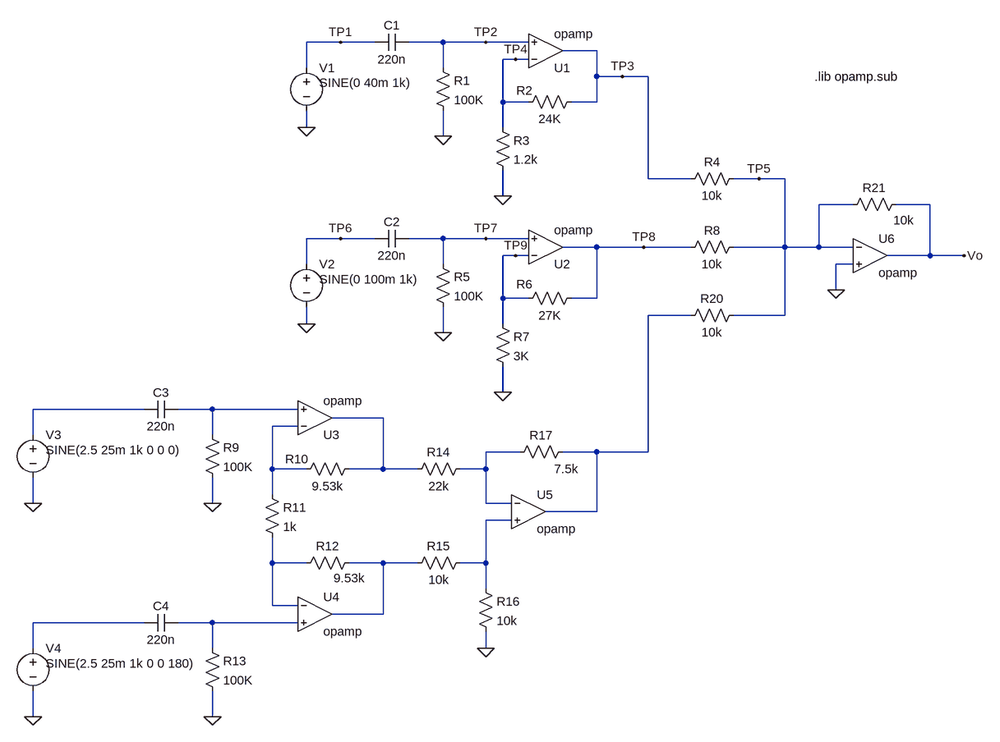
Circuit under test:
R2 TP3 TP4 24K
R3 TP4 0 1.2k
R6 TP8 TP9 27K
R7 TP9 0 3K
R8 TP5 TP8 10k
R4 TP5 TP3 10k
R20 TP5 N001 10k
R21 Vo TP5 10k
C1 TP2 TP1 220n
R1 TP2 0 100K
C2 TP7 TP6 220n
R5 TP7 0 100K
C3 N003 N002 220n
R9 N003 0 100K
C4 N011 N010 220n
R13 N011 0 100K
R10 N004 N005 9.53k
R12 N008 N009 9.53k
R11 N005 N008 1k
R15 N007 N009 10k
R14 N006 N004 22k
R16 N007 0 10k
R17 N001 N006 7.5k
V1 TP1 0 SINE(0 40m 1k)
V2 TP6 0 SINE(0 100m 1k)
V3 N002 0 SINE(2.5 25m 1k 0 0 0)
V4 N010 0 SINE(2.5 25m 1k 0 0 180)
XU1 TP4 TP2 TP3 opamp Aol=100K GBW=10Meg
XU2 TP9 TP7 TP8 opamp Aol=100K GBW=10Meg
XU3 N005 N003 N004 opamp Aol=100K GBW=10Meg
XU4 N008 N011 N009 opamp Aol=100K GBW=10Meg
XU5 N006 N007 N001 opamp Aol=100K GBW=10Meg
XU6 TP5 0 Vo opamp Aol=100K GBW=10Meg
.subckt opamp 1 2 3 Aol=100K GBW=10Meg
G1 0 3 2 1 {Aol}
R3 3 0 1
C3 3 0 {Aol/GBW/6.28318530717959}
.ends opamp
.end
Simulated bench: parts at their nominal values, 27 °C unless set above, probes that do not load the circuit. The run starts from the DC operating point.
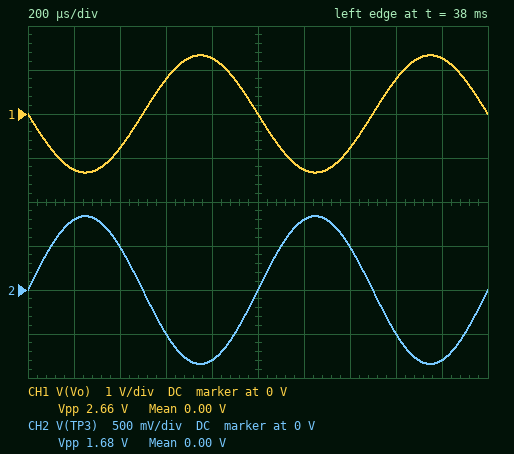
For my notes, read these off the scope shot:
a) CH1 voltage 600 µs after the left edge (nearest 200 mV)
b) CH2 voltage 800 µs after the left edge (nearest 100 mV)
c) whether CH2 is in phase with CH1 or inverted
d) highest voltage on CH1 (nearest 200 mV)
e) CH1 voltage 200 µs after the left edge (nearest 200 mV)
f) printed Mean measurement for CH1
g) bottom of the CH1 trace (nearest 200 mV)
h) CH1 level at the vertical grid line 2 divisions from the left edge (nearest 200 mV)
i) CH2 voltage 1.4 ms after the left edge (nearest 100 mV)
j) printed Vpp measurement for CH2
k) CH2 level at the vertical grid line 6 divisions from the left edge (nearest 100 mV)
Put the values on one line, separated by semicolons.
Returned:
800 mV; -800 mV; inverted; 1.4 V; -1.2 V; 0.00 V; -1.4 V; -800 mV; 500 mV; 1.68 V; 800 mV
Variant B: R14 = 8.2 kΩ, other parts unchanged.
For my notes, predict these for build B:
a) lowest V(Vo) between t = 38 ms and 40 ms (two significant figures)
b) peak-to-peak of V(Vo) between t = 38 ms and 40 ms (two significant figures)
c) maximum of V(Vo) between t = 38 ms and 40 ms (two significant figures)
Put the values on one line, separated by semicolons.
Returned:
-900 mV; 1.8 V; 900 mV
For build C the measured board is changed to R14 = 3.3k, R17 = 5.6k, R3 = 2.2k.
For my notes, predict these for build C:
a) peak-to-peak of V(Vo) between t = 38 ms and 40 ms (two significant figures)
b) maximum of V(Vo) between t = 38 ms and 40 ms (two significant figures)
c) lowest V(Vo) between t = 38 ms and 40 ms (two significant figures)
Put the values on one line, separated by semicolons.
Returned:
100 mV; 51 mV; -51 mV
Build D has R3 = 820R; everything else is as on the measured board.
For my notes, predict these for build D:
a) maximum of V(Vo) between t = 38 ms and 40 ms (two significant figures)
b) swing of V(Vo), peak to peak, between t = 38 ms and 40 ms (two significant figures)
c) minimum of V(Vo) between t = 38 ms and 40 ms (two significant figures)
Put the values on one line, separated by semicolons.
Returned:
1.7 V; 3.4 V; -1.7 V
